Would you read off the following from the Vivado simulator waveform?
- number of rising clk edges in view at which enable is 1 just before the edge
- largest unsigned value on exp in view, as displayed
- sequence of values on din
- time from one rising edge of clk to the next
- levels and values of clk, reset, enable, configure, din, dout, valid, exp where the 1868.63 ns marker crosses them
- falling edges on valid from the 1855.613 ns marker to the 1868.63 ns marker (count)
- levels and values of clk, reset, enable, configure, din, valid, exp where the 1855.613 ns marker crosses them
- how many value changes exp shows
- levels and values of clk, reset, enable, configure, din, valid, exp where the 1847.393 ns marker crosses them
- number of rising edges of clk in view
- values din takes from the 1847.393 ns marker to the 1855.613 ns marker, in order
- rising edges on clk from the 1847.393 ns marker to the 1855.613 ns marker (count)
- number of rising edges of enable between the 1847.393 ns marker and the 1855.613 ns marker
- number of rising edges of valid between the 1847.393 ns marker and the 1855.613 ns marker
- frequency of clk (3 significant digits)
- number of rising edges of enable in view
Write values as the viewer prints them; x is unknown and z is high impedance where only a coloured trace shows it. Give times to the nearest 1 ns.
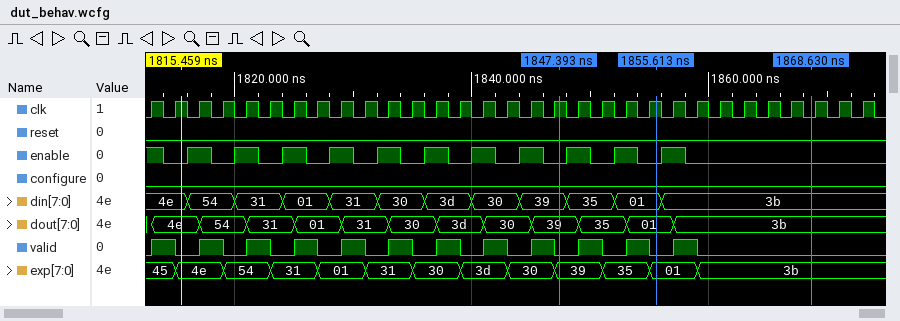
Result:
12
54
4e, 54, 31, 01, 31, 30, 3d, 30, 39, 35, 01, 3b
2 ns
clk=0, reset=0, enable=0, configure=0, din=3b, dout=3b, valid=0, exp=3b
1
clk=1, reset=0, enable=0, configure=0, din=01, valid=0, exp=01
12
clk=1, reset=0, enable=0, configure=0, din=39, valid=0, exp=39
31
39, 35, 01
4
2
2
500 MHz
11
